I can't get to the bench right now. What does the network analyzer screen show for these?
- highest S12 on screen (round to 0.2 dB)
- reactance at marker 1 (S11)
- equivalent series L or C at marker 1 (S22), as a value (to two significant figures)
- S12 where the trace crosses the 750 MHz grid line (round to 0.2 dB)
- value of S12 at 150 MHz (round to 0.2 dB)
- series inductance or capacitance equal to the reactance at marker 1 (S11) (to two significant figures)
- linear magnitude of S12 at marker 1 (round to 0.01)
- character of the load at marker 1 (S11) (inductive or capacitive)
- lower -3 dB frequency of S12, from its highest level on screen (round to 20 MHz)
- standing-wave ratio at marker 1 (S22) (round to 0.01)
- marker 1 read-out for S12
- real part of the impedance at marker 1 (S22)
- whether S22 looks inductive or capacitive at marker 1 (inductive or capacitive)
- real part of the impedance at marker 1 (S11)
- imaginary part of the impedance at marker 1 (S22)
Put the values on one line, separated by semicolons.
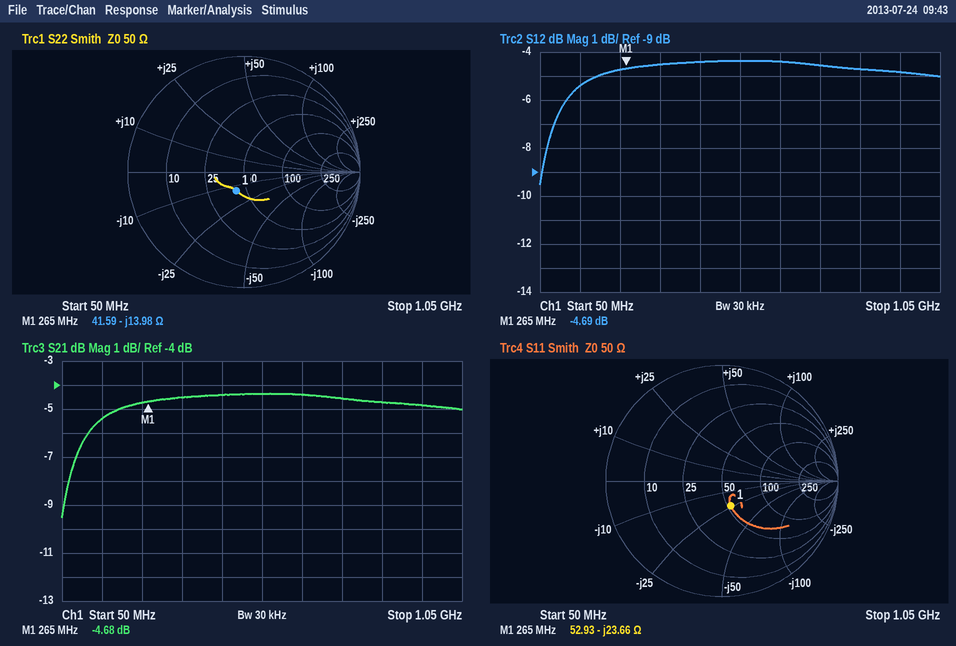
-4.4 dB; -23.66 Ω; 43 pF; -4.6 dB; -5.4 dB; 25 pF; 0.58; capacitive; 80 MHz; 1.43; -4.69 dB; 41.59 Ω; capacitive; 52.93 Ω; -13.98 Ω
